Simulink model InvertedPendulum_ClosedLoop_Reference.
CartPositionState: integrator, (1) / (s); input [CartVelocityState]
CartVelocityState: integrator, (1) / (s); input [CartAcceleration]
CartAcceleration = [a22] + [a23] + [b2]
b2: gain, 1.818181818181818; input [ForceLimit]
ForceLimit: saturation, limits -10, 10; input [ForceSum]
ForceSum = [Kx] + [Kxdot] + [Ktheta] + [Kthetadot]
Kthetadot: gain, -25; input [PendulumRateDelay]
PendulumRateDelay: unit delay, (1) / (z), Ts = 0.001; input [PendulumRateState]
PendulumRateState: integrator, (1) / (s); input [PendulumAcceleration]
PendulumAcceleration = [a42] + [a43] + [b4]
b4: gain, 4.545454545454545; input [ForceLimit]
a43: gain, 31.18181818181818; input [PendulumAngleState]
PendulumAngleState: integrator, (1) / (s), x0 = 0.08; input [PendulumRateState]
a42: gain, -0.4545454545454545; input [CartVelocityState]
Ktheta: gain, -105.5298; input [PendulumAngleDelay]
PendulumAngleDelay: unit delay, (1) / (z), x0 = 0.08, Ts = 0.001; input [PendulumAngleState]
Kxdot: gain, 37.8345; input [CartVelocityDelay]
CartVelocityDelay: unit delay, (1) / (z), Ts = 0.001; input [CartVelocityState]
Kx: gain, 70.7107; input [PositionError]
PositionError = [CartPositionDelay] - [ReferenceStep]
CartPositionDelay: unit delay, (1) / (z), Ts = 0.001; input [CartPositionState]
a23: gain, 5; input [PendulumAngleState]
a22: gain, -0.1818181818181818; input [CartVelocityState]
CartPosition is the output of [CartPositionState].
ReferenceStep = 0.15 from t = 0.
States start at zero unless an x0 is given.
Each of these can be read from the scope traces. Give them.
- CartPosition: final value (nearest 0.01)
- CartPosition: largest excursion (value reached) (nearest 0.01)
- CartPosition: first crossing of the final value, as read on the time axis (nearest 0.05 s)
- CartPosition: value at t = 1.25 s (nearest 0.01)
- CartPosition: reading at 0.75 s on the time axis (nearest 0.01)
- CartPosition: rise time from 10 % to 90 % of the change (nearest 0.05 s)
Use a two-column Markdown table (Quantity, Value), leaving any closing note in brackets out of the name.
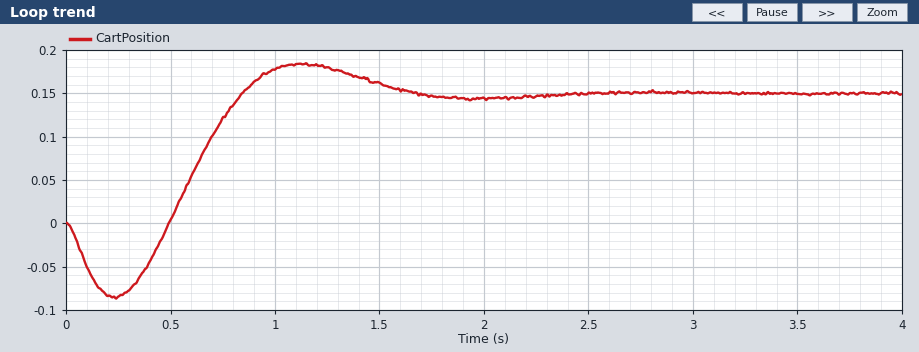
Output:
| Quantity | Value |
|---|---|
| CartPosition: final value | 0.15 |
| CartPosition: largest excursion (value reached) | 0.18 |
| CartPosition: first crossing of the final value, as read on the time axis | 0.85 s |
| CartPosition: value at t = 1.25 s | 0.18 |
| CartPosition: reading at 0.75 s on the time axis | 0.12 |
| CartPosition: rise time from 10 % to 90 % of the change | 0.25 s |
